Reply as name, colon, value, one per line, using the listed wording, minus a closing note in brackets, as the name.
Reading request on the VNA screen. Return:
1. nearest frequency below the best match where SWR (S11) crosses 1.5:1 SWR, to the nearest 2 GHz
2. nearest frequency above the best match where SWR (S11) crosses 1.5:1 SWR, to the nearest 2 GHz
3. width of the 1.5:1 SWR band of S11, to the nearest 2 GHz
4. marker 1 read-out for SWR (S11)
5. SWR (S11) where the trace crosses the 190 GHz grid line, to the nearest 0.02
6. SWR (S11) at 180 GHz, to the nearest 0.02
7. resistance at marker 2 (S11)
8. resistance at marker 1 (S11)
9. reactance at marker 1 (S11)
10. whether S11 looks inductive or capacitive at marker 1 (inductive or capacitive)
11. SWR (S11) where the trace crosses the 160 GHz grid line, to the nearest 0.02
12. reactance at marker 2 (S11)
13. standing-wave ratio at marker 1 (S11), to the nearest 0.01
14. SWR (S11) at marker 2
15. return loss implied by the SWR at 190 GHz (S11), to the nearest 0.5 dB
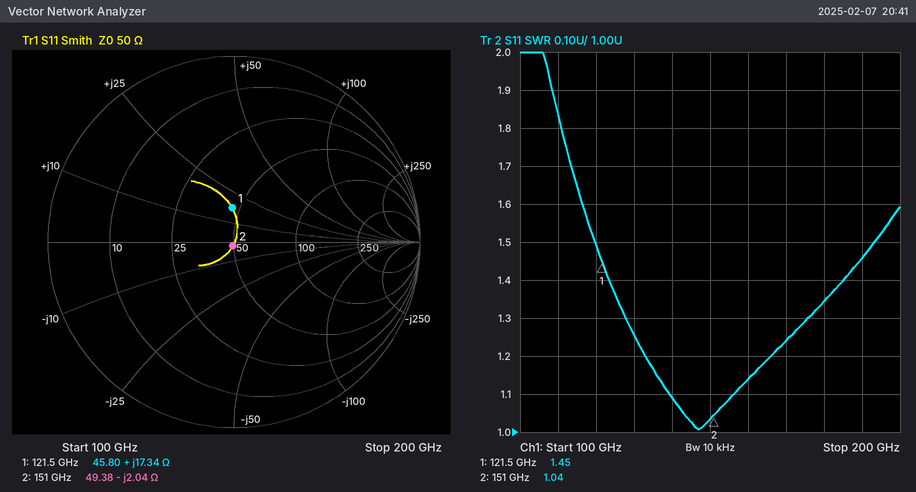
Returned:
nearest frequency below the best match where SWR (S11) crosses 1.5:1 SWR, to the nearest 2 GHz: 120 GHz
nearest frequency above the best match where SWR (S11) crosses 1.5:1 SWR, to the nearest 2 GHz: 194 GHz
width of the 1.5:1 SWR band of S11, to the nearest 2 GHz: 74 GHz
marker 1 read-out for SWR: 1.45
SWR (S11) where the trace crosses the 190 GHz grid line, to the nearest 0.02: 1.46
SWR (S11) at 180 GHz, to the nearest 0.02: 1.34
resistance at marker 2: 49.38 Ω
resistance at marker 1: 45.80 Ω
reactance at marker 1: +17.34 Ω
whether S11 looks inductive or capacitive at marker 1: inductive
SWR (S11) where the trace crosses the 160 GHz grid line, to the nearest 0.02: 1.14
reactance at marker 2: -2.04 Ω
standing-wave ratio at marker 1 (S11), to the nearest 0.01: 1.45
SWR (S11) at marker 2: 1.04
return loss implied by the SWR at 190 GHz (S11), to the nearest 0.5 dB: 14.5 dB
